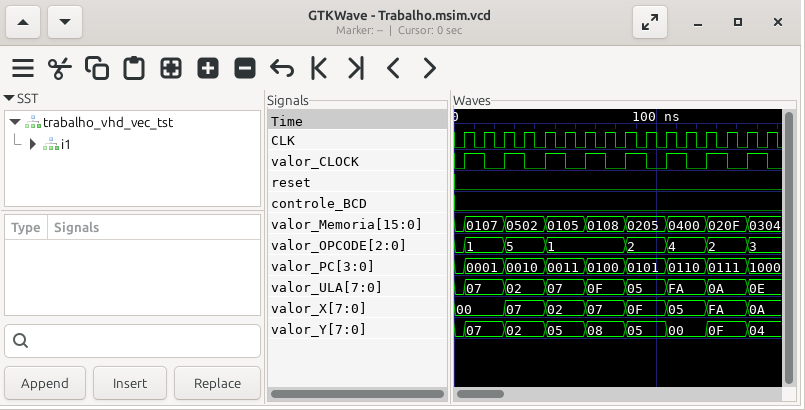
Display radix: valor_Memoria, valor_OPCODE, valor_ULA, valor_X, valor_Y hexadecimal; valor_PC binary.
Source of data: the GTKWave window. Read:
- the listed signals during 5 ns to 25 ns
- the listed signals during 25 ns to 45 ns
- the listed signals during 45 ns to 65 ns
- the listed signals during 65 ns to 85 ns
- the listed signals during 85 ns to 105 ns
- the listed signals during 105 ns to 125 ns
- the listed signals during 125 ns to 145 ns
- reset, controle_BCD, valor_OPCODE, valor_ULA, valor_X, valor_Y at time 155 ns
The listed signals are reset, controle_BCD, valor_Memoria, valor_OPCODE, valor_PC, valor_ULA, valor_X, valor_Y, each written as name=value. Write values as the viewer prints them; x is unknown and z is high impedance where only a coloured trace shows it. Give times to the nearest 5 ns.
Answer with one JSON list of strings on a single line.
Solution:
["reset=0, controle_BCD=0, valor_Memoria=0107, valor_OPCODE=1, valor_PC=0001, valor_ULA=07, valor_X=00, valor_Y=07", "reset=0, controle_BCD=0, valor_Memoria=0502, valor_OPCODE=5, valor_PC=0010, valor_ULA=02, valor_X=07, valor_Y=02", "reset=0, controle_BCD=0, valor_Memoria=0105, valor_OPCODE=1, valor_PC=0011, valor_ULA=07, valor_X=02, valor_Y=05", "reset=0, controle_BCD=0, valor_Memoria=0108, valor_OPCODE=1, valor_PC=0100, valor_ULA=0F, valor_X=07, valor_Y=08", "reset=0, controle_BCD=0, valor_Memoria=0205, valor_OPCODE=2, valor_PC=0101, valor_ULA=05, valor_X=0F, valor_Y=05", "reset=0, controle_BCD=0, valor_Memoria=0400, valor_OPCODE=4, valor_PC=0110, valor_ULA=FA, valor_X=05, valor_Y=00", "reset=0, controle_BCD=0, valor_Memoria=020F, valor_OPCODE=2, valor_PC=0111, valor_ULA=0A, valor_X=FA, valor_Y=0F", "reset=0, controle_BCD=0, valor_OPCODE=3, valor_ULA=0E, valor_X=0A, valor_Y=04"]
